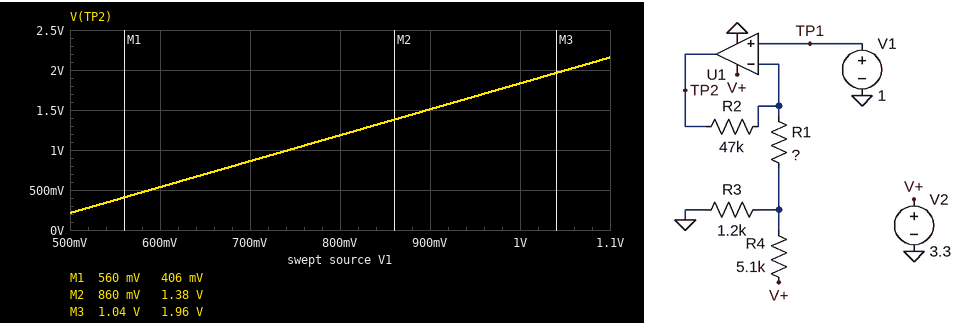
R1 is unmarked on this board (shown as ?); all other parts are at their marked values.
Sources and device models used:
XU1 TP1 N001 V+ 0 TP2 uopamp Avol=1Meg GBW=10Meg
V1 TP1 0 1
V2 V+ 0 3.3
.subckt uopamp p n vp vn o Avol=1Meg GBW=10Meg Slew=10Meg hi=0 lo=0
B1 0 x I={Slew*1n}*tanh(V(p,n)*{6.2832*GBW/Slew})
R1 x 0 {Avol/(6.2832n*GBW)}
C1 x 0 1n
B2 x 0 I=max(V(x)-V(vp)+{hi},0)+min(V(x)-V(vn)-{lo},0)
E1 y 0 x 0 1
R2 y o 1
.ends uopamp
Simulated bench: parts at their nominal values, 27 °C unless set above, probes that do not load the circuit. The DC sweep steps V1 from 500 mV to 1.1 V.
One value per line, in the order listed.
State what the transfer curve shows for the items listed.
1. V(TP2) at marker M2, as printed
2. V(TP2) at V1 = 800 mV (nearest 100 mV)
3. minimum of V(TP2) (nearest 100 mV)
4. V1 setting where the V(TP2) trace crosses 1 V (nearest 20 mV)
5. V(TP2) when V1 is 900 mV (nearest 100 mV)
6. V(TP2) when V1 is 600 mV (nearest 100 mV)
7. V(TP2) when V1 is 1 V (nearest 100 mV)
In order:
1.38 V
1.2 V
200 mV
740 mV
1.5 V
500 mV
1.8 V
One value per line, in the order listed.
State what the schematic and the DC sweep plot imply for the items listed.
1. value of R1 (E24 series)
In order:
20 kΩ
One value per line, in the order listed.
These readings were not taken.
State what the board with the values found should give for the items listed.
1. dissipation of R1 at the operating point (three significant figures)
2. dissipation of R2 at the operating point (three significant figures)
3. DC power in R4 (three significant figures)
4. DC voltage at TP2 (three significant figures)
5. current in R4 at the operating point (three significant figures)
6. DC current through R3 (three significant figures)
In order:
6.27 µW
14.7 µW
1.38 mW
1.83 V
520 µA
538 µA
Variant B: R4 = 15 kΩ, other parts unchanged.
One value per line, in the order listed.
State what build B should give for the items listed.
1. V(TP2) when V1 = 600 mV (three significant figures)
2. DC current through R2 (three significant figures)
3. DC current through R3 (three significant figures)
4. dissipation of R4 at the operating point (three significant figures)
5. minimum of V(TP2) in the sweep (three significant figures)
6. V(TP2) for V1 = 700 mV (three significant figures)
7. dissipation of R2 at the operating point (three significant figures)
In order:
1.39 V
35.8 µA
237 µA
606 µW
1.07 V
1.71 V
60.2 µW
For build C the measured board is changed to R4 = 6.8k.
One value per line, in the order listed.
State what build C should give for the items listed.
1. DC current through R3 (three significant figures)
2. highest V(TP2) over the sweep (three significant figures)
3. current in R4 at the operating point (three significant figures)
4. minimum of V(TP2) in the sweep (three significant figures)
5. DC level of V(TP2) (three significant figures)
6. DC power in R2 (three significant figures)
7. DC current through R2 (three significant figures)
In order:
433 µA
2.45 V
409 µA
511 mV
2.13 V
27.1 µW
24.0 µA
